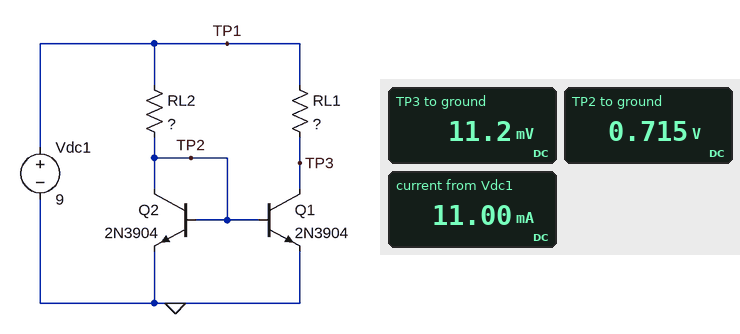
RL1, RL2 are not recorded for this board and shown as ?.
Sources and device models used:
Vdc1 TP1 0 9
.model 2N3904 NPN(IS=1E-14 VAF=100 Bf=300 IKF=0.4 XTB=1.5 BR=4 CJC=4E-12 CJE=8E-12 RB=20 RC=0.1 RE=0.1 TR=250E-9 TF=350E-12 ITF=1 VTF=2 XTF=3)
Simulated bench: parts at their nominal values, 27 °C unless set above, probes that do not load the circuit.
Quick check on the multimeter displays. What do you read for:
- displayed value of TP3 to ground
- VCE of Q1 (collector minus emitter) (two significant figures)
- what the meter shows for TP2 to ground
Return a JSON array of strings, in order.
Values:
["11.2 mV", "11 mV", "0.715 V"]
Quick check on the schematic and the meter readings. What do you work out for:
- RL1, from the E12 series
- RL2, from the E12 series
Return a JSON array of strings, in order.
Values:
["10 kΩ", "820 Ω"]
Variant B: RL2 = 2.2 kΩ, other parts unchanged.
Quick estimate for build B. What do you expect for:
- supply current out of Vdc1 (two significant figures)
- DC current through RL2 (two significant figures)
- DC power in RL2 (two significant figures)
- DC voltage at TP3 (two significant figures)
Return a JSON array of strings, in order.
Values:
["4.7 mA", "3.8 mA", "31 mW", "17 mV"]
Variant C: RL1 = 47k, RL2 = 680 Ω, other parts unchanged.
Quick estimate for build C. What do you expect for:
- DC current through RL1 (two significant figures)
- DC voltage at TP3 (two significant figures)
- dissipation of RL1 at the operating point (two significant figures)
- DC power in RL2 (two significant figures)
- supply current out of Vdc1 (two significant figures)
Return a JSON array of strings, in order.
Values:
["190 µA", "7.0 mV", "1.7 mW", "100 mW", "12 mA"]
